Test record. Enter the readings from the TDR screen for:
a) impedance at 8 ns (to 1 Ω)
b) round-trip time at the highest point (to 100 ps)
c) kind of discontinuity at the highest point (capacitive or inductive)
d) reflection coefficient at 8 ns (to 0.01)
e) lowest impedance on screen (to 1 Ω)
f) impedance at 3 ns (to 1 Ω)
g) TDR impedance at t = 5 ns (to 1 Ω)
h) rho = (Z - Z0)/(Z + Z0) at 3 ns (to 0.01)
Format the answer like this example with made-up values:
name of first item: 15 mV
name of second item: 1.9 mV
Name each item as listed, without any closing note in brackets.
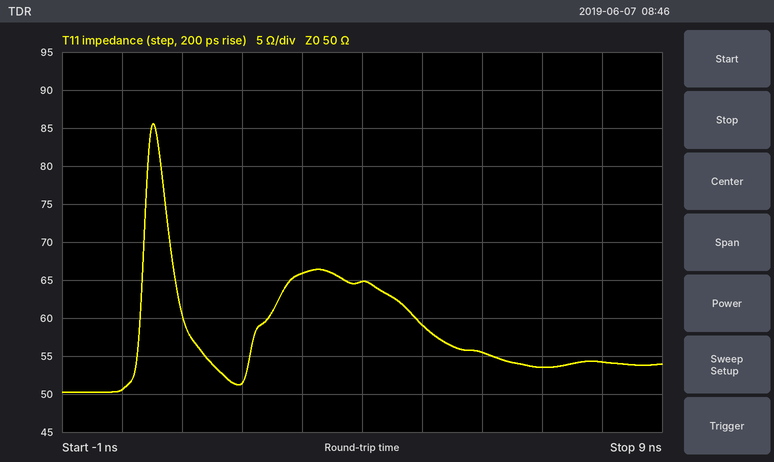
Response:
impedance at 8 ns: 54 Ω
round-trip time at the highest point: 500 ps
kind of discontinuity at the highest point: inductive
reflection coefficient at 8 ns: +0.04
lowest impedance on screen: 50 Ω
impedance at 3 ns: 66 Ω
TDR impedance at t = 5 ns: 59 Ω
rho = (Z - Z0)/(Z + Z0) at 3 ns: +0.14
